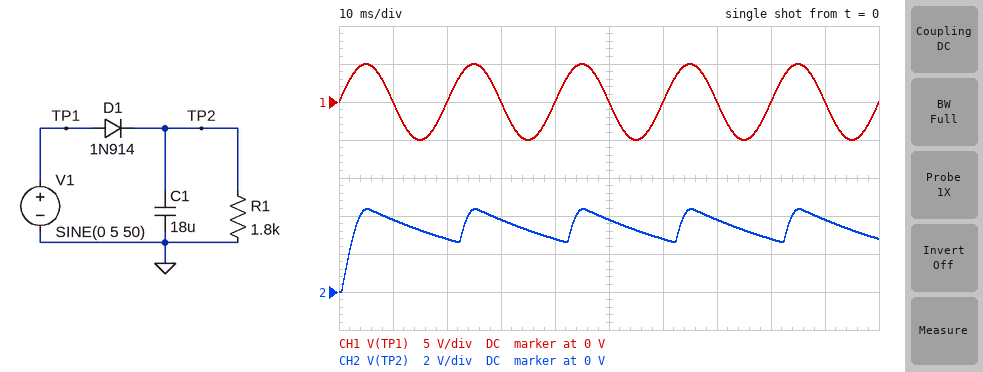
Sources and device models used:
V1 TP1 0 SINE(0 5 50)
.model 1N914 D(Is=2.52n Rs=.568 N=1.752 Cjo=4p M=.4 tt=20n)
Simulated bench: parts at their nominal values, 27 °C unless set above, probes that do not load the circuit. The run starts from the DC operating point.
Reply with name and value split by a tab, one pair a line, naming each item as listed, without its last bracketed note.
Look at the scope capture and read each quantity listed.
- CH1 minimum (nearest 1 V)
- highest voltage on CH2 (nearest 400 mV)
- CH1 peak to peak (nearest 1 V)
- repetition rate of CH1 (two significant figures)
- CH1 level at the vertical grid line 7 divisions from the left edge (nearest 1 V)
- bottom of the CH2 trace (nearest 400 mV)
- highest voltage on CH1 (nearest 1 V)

CH1 minimum	-5 V
highest voltage on CH2	4.4 V
CH1 peak to peak	10 V
repetition rate of CH1	50 Hz
CH1 level at the vertical grid line 7 divisions from the left edge	0 V
bottom of the CH2 trace	0 V
highest voltage on CH1	5 V
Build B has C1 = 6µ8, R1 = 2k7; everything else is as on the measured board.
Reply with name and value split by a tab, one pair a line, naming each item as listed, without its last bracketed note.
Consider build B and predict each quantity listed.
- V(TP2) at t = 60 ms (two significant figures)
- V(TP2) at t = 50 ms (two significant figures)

V(TP2) at t = 60 ms	2.0 V
V(TP2) at t = 50 ms	3.4 V
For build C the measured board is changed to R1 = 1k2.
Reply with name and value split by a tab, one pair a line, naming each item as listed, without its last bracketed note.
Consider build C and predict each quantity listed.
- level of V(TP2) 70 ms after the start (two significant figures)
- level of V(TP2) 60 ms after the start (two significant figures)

level of V(TP2) 70 ms after the start	3.5 V
level of V(TP2) 60 ms after the start	2.2 V
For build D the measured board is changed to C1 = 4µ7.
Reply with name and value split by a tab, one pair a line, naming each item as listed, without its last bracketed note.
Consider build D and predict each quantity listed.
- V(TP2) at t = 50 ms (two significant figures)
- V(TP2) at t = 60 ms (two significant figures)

V(TP2) at t = 50 ms	2.6 V
V(TP2) at t = 60 ms	810 mV
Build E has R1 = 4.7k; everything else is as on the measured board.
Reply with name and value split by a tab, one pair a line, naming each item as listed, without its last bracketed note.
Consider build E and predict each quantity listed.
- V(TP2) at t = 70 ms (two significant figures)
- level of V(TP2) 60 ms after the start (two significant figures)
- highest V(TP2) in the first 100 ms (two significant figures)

V(TP2) at t = 70 ms	4.2 V
level of V(TP2) 60 ms after the start	3.7 V
highest V(TP2) in the first 100 ms	4.4 V
